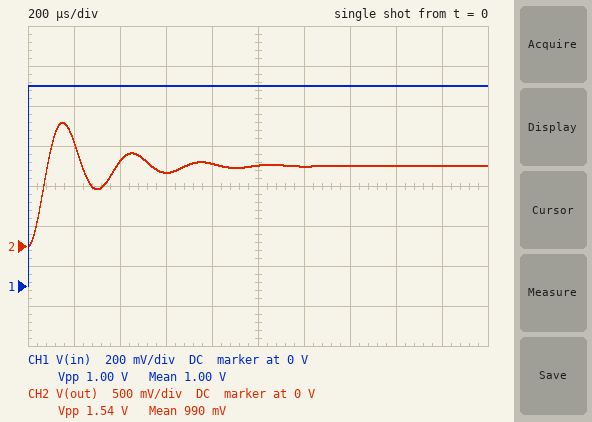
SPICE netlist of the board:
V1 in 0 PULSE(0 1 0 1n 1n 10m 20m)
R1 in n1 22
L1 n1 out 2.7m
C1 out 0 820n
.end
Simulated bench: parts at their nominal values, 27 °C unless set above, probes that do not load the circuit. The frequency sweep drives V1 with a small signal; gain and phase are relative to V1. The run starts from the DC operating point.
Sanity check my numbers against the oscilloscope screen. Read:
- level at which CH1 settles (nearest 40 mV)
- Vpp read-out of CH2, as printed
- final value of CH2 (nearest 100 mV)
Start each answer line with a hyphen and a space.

- 1.00 V
- 1.54 V
- 1.0 V
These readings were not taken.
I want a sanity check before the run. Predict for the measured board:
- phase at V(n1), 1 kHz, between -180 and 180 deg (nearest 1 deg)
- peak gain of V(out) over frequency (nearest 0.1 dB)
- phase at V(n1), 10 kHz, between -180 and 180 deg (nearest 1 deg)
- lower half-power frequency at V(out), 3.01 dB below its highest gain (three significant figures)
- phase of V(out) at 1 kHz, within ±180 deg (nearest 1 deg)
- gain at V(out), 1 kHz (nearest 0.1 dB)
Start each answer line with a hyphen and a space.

- -7 deg
- 8.5 dB
- 8 deg
- 2.51 kHz
- -7 deg
- 0.7 dB
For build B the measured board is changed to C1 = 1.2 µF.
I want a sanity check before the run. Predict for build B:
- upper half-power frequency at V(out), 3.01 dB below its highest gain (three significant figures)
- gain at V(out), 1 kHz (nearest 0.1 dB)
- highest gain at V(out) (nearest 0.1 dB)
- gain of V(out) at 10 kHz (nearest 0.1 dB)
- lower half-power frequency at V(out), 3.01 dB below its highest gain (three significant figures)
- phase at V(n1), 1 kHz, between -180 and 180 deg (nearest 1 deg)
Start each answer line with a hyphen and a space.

- 3.24 kHz
- 1.0 dB
- 6.9 dB
- -21.5 dB
- 1.86 kHz
- -11 deg
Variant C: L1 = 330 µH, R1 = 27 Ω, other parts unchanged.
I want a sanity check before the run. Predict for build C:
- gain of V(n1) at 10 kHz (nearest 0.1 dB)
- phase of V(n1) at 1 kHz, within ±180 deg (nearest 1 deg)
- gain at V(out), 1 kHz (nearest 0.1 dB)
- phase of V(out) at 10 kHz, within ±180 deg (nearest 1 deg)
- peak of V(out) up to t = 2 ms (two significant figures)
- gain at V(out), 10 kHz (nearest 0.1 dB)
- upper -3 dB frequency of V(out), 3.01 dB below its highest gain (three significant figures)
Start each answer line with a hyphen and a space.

- -26.2 dB
- -8 deg
- 0 dB
- -93 deg
- 1.1 V
- -2.9 dB
- 10.1 kHz
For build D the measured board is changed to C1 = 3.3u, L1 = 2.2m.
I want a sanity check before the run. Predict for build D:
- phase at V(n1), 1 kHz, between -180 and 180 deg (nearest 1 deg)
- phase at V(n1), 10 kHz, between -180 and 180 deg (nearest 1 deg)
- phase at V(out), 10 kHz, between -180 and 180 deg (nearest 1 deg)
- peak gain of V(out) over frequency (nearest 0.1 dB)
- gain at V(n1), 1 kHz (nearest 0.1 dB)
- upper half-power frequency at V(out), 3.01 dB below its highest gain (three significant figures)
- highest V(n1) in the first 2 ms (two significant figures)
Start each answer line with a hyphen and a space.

- -33 deg
- 9 deg
- -171 deg
- 2.3 dB
- -1.5 dB
- 2.22 kHz
- 1.1 V
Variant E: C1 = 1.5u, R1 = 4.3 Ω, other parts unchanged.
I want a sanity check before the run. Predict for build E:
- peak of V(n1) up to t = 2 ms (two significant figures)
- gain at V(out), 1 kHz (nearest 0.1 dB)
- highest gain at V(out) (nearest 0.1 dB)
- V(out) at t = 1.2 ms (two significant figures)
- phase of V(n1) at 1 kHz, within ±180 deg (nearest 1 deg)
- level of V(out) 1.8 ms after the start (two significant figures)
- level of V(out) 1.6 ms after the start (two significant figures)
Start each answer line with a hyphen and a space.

- 1.1 V
- 1.5 dB
- 19.9 dB
- 620 mV
- -3 deg
- 1.2 V
- 720 mV
